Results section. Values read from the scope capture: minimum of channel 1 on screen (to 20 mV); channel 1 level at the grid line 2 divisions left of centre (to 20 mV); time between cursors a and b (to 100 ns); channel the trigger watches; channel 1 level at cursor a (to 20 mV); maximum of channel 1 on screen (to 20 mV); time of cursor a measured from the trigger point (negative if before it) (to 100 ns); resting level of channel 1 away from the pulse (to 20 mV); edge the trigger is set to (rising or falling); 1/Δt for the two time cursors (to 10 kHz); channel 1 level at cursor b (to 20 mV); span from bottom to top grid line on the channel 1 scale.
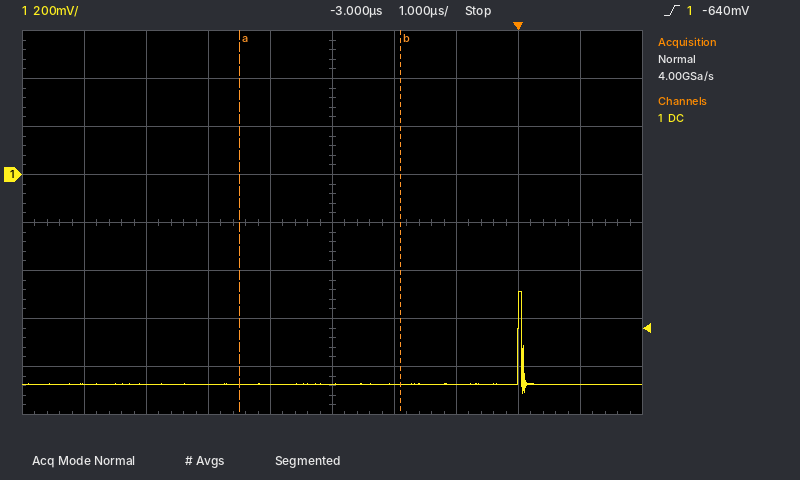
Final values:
-920 mV
-880 mV
2.6 µs
channel 1
-880 mV
-480 mV
-4.5 µs
-880 mV
rising
380 kHz
-880 mV
1.6 V
